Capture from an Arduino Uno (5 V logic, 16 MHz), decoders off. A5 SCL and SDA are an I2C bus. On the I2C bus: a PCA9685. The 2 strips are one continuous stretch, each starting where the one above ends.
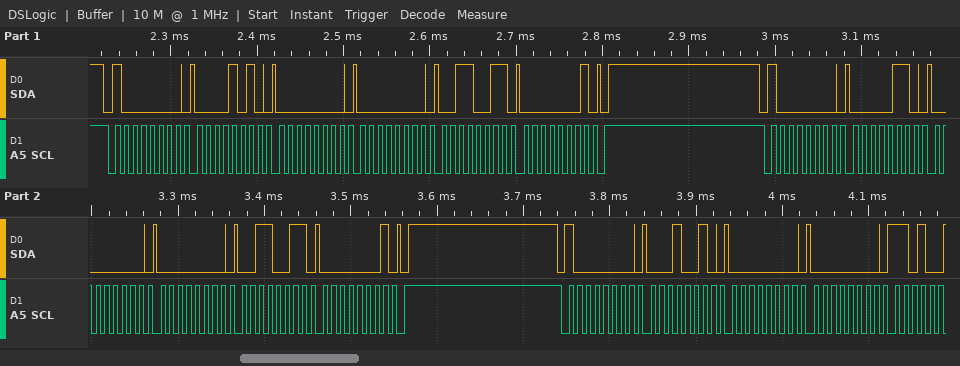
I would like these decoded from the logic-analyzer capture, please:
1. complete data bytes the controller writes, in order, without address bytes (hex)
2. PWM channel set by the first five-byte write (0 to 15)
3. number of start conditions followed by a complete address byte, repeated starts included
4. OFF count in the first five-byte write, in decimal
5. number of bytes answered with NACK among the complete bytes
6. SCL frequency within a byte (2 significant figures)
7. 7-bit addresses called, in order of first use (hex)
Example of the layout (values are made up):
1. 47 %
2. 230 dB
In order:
1. 0A 00 00 33 01 06 00 00 33 01 12 00 00
2. 1
3. 3
4. 307
5. 0
6. 100 kHz
7. 0x40
